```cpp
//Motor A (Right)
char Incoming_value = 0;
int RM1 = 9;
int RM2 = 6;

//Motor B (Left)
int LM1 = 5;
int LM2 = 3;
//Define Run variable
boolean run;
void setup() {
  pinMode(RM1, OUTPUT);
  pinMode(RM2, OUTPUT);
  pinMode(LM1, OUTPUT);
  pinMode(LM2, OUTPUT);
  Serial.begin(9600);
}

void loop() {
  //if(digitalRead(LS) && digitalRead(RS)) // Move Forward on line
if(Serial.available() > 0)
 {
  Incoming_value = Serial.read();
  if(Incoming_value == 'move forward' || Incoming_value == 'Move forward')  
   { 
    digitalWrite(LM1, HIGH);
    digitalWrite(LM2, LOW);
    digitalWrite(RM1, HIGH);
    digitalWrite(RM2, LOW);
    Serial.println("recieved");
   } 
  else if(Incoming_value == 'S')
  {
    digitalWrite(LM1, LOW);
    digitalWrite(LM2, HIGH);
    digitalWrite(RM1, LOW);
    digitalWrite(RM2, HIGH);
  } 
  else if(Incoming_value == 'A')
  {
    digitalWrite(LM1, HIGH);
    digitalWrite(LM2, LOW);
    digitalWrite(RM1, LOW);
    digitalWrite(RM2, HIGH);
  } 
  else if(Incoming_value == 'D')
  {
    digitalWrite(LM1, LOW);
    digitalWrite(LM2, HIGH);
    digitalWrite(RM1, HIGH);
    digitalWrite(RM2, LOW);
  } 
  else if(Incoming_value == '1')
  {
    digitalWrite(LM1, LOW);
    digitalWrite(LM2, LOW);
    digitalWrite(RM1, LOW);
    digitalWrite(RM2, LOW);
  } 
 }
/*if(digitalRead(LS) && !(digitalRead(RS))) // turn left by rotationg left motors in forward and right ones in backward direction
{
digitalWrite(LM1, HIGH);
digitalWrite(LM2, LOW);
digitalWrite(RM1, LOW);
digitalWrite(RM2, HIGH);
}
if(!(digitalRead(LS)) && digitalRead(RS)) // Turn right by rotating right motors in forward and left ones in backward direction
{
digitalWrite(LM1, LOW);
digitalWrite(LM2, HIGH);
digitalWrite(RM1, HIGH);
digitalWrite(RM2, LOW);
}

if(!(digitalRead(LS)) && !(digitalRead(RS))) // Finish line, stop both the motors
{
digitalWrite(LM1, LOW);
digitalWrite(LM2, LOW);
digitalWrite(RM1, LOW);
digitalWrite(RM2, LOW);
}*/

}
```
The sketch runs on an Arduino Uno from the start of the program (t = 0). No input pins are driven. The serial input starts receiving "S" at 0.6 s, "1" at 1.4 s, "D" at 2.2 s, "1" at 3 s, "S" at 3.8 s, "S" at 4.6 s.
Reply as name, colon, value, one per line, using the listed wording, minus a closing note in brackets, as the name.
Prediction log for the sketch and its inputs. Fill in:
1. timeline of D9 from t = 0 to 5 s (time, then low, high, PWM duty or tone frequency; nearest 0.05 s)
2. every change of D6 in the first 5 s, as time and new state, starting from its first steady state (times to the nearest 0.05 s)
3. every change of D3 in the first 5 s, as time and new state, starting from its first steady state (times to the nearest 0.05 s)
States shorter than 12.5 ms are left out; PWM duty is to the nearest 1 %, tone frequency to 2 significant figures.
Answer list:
timeline of D9 from t = 0 to 5 s: 0 s low; 2.2 s high; 3 s low
every change of D6 in the first 5 s, as time and new state, starting from its first steady state: 0 s low; 0.6 s high; 1.4 s low; 3.8 s high
every change of D3 in the first 5 s, as time and new state, starting from its first steady state: 0 s low; 0.6 s high; 1.4 s low; 2.2 s high; 3 s low; 3.8 s high
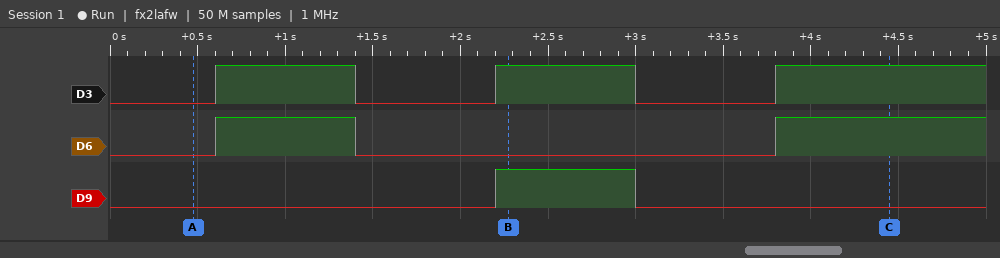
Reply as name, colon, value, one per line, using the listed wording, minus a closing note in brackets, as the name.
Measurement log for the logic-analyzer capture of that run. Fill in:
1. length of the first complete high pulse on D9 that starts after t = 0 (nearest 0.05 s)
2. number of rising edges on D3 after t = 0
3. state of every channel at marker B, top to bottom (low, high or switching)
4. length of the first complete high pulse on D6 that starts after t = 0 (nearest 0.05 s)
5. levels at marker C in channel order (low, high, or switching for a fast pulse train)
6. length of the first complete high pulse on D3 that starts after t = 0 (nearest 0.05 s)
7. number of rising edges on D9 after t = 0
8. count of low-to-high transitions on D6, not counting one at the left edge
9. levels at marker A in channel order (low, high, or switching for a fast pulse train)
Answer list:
length of the first complete high pulse on D9 that starts after t = 0: 0.80 s
number of rising edges on D3 after t = 0: 3
state of every channel at marker B, top to bottom: D3 high, D6 low, D9 high
length of the first complete high pulse on D6 that starts after t = 0: 0.80 s
levels at marker C in channel order: D3 high, D6 high, D9 low
length of the first complete high pulse on D3 that starts after t = 0: 0.80 s
number of rising edges on D9 after t = 0: 1
count of low-to-high transitions on D6, not counting one at the left edge: 2
levels at marker A in channel order: D3 low, D6 low, D9 low
